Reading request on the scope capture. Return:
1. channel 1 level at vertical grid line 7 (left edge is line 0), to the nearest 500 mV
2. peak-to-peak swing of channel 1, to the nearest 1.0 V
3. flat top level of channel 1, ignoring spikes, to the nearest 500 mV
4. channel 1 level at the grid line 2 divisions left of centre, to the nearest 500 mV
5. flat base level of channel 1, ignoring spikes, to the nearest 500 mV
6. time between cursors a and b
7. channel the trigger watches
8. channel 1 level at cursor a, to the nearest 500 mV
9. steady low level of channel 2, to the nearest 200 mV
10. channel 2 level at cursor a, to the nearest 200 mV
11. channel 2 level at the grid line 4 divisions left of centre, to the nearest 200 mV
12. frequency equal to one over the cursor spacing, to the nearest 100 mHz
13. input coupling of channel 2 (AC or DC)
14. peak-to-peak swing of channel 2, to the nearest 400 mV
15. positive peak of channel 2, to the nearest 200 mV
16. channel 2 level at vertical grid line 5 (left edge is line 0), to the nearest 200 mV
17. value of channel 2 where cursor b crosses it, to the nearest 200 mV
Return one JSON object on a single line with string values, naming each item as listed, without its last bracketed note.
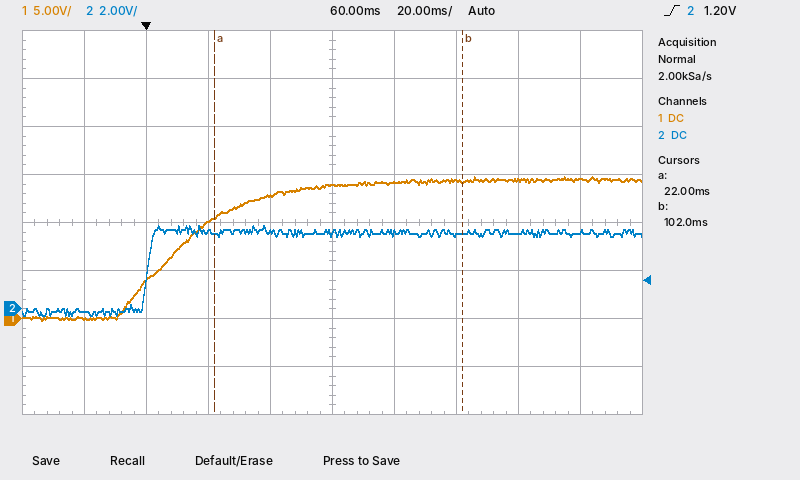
{"channel 1 level at vertical grid line 7 (left edge is line 0), to the nearest 500 mV": "14.5 V", "peak-to-peak swing of channel 1, to the nearest 1.0 V": "15.0 V", "flat top level of channel 1, ignoring spikes, to the nearest 500 mV": "14.5 V", "channel 1 level at the grid line 2 divisions left of centre, to the nearest 500 mV": "10.0 V", "flat base level of channel 1, ignoring spikes, to the nearest 500 mV": "0.0 V", "time between cursors a and b": "80 ms", "channel the trigger watches": "channel 2", "channel 1 level at cursor a, to the nearest 500 mV": "10.5 V", "steady low level of channel 2, to the nearest 200 mV": "-200 mV", "channel 2 level at cursor a, to the nearest 200 mV": "3.2 V", "channel 2 level at the grid line 4 divisions left of centre, to the nearest 200 mV": "-200 mV", "frequency equal to one over the cursor spacing, to the nearest 100 mHz": "12.5 Hz", "input coupling of channel 2": "DC", "peak-to-peak swing of channel 2, to the nearest 400 mV": "3.6 V", "positive peak of channel 2, to the nearest 200 mV": "3.4 V", "channel 2 level at vertical grid line 5 (left edge is line 0), to the nearest 200 mV": "3.2 V", "value of channel 2 where cursor b crosses it, to the nearest 200 mV": "3.2 V"}
